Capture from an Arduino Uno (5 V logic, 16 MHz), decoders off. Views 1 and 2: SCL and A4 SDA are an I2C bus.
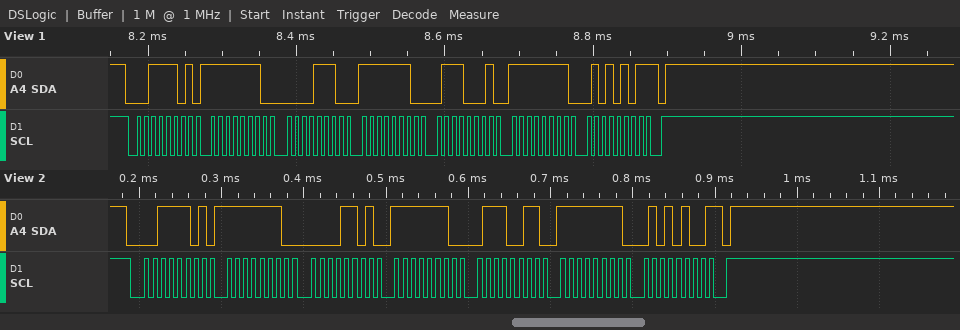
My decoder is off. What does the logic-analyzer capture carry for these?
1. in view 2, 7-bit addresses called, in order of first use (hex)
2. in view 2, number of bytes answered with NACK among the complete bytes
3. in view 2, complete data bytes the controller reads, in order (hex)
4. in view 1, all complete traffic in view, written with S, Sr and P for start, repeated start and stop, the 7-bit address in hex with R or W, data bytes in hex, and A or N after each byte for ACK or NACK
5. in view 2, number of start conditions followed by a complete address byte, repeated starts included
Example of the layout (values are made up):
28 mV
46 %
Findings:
0x1E
1
FE 0D FE 73 FF 54
S 1ER A FE A 0E A FE A 71 A FF A 55 N P
1
